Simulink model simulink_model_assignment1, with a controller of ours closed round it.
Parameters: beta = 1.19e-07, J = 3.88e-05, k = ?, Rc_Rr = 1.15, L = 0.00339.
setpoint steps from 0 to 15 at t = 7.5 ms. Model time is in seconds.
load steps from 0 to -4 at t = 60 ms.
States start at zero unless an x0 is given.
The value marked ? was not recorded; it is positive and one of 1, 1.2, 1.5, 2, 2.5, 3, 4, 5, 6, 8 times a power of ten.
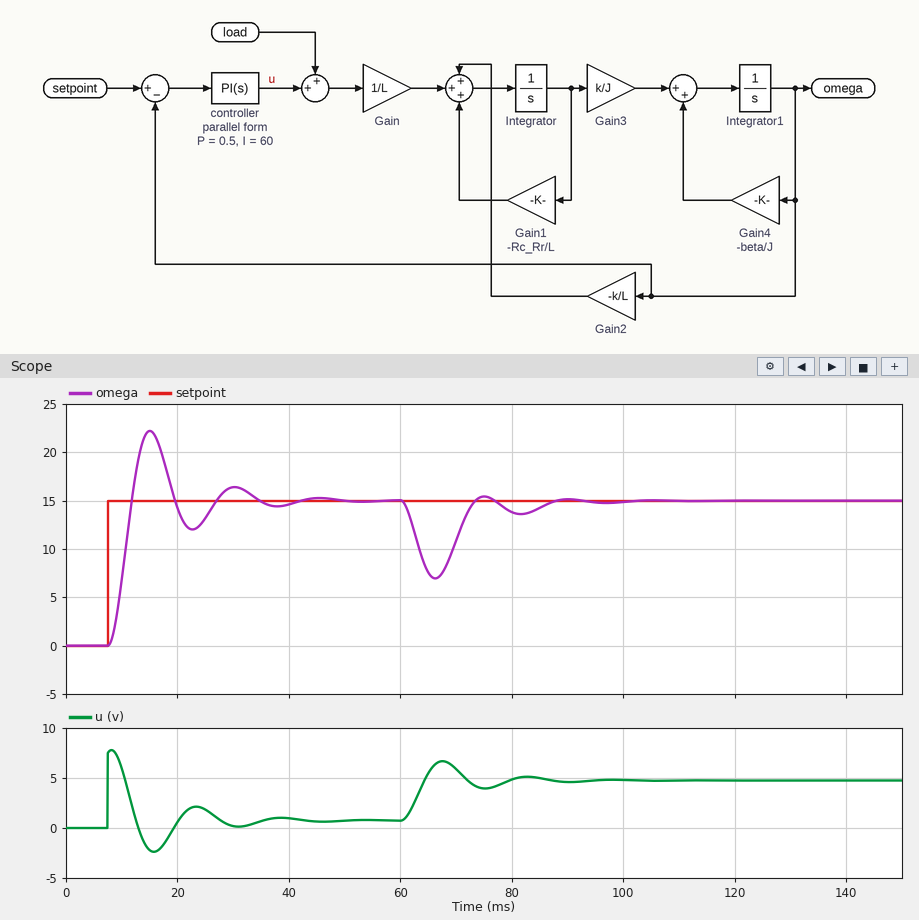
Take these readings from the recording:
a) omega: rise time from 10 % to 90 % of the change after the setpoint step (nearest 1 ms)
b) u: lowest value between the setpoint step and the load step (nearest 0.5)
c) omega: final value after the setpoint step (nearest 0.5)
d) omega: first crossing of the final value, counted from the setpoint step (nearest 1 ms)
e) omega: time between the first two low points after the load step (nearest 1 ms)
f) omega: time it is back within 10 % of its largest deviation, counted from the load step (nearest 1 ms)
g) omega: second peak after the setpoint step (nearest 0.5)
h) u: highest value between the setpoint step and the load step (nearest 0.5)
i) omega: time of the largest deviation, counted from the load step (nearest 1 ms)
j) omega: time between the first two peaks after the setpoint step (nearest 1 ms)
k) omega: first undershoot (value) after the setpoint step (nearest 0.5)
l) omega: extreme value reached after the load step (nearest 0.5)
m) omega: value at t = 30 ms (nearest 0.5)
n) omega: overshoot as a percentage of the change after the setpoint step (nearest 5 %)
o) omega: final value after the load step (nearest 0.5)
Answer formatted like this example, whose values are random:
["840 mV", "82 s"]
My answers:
["3 ms", "-2.5", "15.0", "4 ms", "15 ms", "25 ms", "16.5", "8.0", "6 ms", "15 ms", "12.0", "7.0", "16.5", "50 %", "15.0"]
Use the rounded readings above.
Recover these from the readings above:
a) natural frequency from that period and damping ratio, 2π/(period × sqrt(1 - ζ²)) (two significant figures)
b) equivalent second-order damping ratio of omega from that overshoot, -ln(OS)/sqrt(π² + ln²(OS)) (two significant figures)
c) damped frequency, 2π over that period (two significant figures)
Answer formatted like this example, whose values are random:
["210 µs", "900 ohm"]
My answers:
["0.43 rad/ms", "0.22", "0.42 rad/ms"]
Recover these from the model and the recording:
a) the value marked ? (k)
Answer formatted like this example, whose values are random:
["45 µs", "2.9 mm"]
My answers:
["0.05"]
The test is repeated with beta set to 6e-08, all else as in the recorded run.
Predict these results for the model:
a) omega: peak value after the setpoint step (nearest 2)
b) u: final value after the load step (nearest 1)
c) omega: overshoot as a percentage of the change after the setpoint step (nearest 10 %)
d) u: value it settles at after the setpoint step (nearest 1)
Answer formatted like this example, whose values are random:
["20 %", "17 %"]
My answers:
["22", "5", "50 %", "1"]
